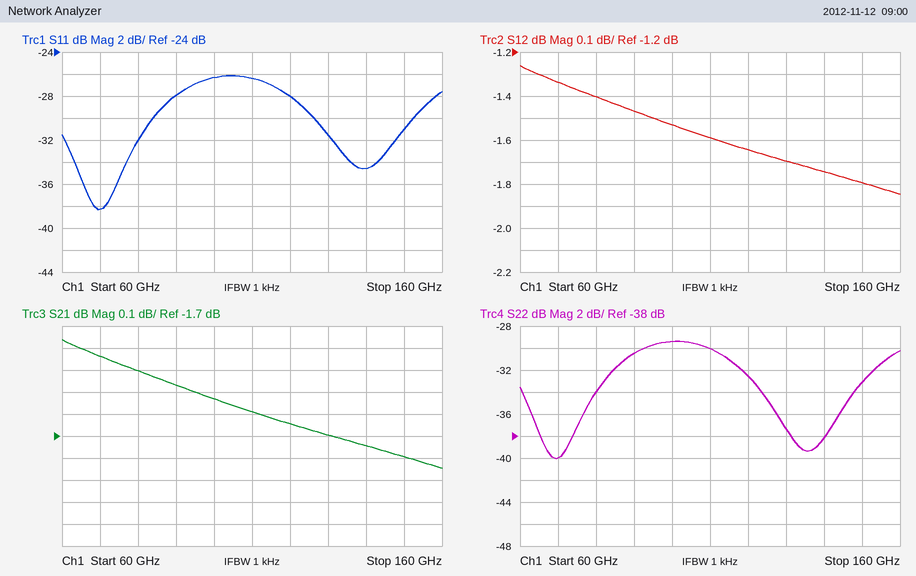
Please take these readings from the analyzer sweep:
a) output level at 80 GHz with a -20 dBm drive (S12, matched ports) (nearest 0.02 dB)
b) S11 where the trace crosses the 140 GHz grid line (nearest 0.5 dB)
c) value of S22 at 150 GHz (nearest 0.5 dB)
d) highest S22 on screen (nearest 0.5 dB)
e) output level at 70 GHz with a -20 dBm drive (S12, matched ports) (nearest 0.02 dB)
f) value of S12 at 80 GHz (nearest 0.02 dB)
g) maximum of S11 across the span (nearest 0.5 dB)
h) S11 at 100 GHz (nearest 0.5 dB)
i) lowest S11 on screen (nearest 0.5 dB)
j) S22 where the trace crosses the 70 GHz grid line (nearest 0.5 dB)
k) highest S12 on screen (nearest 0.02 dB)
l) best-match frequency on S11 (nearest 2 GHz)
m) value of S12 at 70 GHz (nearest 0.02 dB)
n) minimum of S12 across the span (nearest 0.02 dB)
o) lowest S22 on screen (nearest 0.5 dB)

-21.40 dBm
-34.5 dB
-33.0 dB
-29.5 dB
-21.34 dBm
-1.40 dB
-26.0 dB
-26.5 dB
-38.5 dB
-40.0 dB
-1.26 dB
70 GHz
-1.34 dB
-1.84 dB
-40.0 dB
